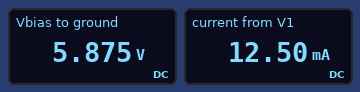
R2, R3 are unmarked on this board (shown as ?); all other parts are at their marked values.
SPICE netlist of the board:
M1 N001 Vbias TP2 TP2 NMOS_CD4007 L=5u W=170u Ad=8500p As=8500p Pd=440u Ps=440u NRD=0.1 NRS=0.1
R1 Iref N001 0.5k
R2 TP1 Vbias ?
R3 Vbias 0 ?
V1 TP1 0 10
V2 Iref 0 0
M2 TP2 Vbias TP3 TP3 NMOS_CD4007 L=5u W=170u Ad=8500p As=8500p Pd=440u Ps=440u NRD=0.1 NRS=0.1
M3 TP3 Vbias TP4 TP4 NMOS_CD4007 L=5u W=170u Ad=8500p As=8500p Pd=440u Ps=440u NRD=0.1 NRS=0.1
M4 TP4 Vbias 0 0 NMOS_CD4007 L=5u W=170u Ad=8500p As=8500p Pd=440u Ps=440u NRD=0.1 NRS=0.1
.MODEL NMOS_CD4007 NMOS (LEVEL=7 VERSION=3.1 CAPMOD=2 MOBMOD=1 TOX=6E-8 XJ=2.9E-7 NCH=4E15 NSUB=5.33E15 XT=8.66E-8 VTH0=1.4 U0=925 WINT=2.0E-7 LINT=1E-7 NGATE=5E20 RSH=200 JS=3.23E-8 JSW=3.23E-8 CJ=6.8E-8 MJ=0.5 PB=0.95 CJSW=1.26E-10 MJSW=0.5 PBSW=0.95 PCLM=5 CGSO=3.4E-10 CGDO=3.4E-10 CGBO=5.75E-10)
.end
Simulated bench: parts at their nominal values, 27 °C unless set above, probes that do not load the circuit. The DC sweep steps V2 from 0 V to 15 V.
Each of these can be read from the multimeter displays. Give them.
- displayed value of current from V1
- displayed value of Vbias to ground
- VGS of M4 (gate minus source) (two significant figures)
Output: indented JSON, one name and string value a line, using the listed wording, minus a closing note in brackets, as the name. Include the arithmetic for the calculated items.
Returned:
{
  "displayed value of current from V1": "12.50 mA",
  "displayed value of Vbias to ground": "5.875 V",
  "VGS of M4 (gate minus source)": "5.875 V = 5.9 V"
}
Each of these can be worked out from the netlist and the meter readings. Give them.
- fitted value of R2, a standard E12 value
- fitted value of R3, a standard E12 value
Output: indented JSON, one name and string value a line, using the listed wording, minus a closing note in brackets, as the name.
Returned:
{
  "fitted value of R2, a standard E12 value": "330 Ω",
  "fitted value of R3, a standard E12 value": "470 Ω"
}
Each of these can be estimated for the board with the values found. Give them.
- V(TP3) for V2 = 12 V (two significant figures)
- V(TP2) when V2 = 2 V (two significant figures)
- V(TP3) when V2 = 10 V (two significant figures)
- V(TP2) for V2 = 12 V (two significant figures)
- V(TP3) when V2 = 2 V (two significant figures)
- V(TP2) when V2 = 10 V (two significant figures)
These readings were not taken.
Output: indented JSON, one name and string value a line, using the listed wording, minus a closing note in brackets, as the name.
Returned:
{
  "V(TP3) for V2 = 12 V": "1.3 V",
  "V(TP2) when V2 = 2 V": "930 mV",
  "V(TP3) when V2 = 10 V": "1.3 V",
  "V(TP2) for V2 = 12 V": "2.2 V",
  "V(TP3) when V2 = 2 V": "600 mV",
  "V(TP2) when V2 = 10 V": "2.2 V"
}
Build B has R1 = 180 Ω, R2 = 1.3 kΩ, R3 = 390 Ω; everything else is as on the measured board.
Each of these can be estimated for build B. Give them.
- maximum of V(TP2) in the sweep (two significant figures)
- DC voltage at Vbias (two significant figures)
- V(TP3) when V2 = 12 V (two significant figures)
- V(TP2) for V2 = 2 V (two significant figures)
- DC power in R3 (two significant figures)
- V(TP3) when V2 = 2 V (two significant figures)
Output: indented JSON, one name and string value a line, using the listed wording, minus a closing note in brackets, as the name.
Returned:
{
  "maximum of V(TP2) in the sweep": "520 mV",
  "DC voltage at Vbias": "2.3 V",
  "V(TP3) when V2 = 12 V": "280 mV",
  "V(TP2) for V2 = 2 V": "440 mV",
  "DC power in R3": "14 mW",
  "V(TP3) when V2 = 2 V": "260 mV"
}
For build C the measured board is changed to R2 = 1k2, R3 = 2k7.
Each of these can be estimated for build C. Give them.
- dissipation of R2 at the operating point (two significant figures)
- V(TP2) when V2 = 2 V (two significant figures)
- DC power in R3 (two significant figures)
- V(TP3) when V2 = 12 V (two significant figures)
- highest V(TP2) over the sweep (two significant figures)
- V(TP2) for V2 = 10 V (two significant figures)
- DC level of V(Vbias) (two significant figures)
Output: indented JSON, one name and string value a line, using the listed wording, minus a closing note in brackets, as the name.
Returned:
{
  "dissipation of R2 at the operating point": "7.9 mW",
  "V(TP2) when V2 = 2 V": "880 mV",
  "DC power in R3": "18 mW",
  "V(TP3) when V2 = 12 V": "1.6 V",
  "highest V(TP2) over the sweep": "2.8 V",
  "V(TP2) for V2 = 10 V": "2.7 V",
  "DC level of V(Vbias)": "6.9 V"
}
